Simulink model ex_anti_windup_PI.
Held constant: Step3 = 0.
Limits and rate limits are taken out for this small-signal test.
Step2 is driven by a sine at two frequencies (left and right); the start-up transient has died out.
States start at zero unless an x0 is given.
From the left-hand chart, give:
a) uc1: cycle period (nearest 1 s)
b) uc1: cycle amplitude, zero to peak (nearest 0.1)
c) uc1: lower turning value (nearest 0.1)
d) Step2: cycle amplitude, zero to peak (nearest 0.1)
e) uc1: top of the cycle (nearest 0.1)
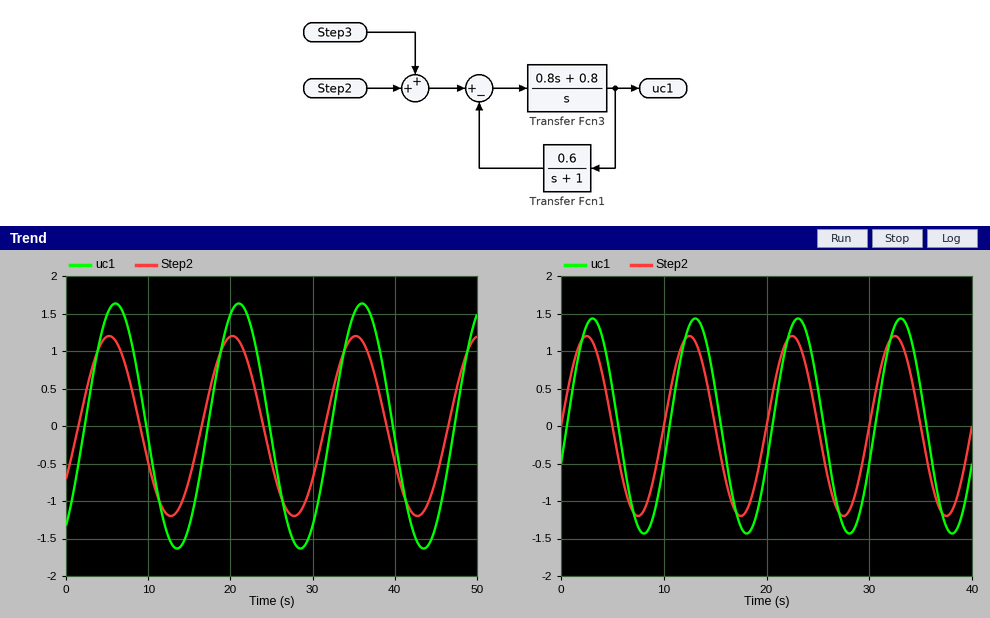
15 s
1.6
-1.6
1.2
1.6
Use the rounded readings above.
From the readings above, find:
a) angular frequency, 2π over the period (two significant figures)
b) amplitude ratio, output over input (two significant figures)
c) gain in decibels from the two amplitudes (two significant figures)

0.42 rad/s
1.3
2.5 dB
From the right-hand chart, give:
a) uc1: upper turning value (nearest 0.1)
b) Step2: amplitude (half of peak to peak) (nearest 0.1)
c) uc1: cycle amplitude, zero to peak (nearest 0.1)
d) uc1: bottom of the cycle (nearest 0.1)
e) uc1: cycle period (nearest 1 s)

1.4
1.2
1.4
-1.4
10 s
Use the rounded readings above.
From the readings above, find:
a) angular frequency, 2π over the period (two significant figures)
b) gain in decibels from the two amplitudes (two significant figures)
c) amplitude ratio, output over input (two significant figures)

0.63 rad/s
1.3 dB
1.2
